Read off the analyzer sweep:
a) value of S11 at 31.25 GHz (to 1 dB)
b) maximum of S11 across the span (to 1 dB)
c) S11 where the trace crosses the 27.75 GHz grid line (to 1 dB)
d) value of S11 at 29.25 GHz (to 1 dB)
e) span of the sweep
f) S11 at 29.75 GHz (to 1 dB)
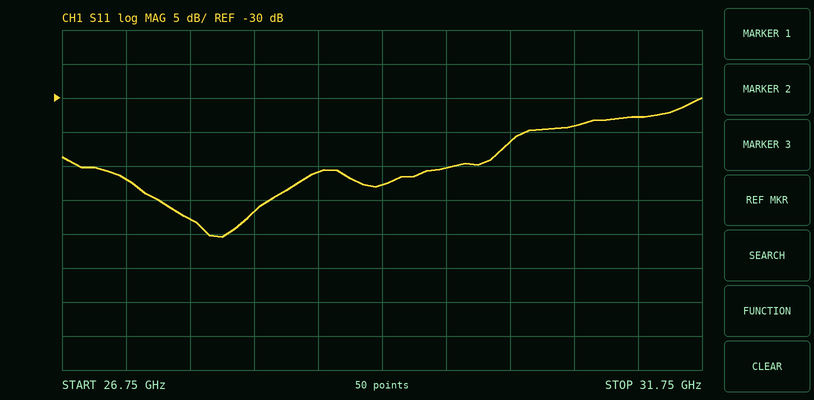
-33 dB
-30 dB
-48 dB
-43 dB
5 GHz
-40 dB
